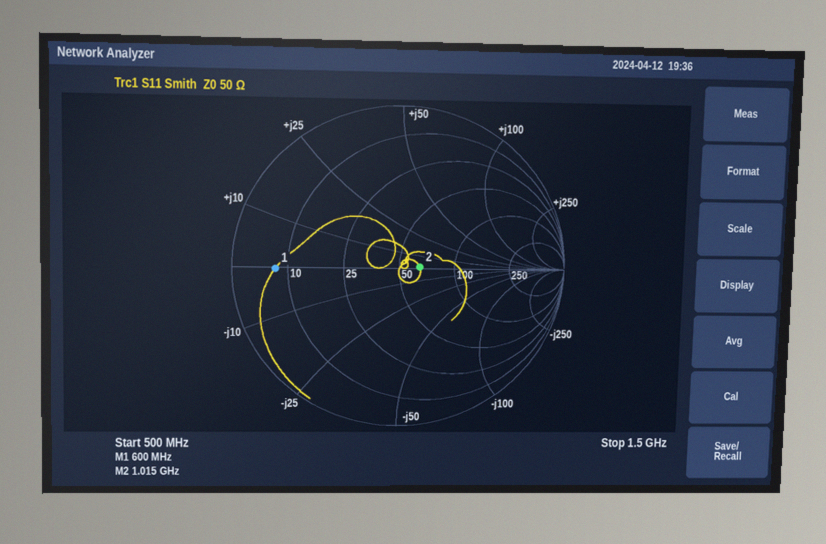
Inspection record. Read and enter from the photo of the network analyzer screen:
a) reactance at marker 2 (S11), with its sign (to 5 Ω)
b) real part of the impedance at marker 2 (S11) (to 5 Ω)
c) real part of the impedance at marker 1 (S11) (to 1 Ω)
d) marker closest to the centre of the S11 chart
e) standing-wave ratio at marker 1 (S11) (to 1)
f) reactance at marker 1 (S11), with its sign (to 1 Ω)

0 Ω
65 Ω
7 Ω
marker 2
7
0 Ω
